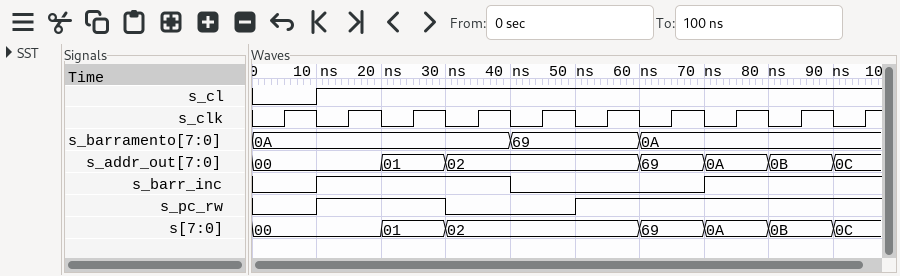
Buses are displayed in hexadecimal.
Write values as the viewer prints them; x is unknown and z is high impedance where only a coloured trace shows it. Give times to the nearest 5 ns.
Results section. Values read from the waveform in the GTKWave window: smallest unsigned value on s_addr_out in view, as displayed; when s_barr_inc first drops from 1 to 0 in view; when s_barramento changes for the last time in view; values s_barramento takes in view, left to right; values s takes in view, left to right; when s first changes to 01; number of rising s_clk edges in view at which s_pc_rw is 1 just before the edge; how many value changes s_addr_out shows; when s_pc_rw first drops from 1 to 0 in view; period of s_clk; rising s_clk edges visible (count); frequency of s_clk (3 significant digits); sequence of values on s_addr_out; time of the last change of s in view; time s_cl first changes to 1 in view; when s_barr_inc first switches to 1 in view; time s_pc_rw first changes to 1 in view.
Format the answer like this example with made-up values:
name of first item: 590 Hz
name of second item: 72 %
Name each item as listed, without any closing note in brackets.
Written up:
smallest unsigned value on s_addr_out in view, as displayed: 00
when s_barr_inc first drops from 1 to 0 in view: 40 ns
when s_barramento changes for the last time in view: 60 ns
values s_barramento takes in view, left to right: 0A, 69, 0A
values s takes in view, left to right: 00, 01, 02, 69, 0A, 0B, 0C
when s first changes to 01: 20 ns
number of rising s_clk edges in view at which s_pc_rw is 1 just before the edge: 7
how many value changes s_addr_out shows: 6
when s_pc_rw first drops from 1 to 0 in view: 30 ns
period of s_clk: 10 ns
rising s_clk edges visible: 10
frequency of s_clk: 100 MHz
sequence of values on s_addr_out: 00, 01, 02, 69, 0A, 0B, 0C
time of the last change of s in view: 90 ns
time s_cl first changes to 1 in view: 10 ns
when s_barr_inc first switches to 1 in view: 10 ns
time s_pc_rw first changes to 1 in view: 10 ns
